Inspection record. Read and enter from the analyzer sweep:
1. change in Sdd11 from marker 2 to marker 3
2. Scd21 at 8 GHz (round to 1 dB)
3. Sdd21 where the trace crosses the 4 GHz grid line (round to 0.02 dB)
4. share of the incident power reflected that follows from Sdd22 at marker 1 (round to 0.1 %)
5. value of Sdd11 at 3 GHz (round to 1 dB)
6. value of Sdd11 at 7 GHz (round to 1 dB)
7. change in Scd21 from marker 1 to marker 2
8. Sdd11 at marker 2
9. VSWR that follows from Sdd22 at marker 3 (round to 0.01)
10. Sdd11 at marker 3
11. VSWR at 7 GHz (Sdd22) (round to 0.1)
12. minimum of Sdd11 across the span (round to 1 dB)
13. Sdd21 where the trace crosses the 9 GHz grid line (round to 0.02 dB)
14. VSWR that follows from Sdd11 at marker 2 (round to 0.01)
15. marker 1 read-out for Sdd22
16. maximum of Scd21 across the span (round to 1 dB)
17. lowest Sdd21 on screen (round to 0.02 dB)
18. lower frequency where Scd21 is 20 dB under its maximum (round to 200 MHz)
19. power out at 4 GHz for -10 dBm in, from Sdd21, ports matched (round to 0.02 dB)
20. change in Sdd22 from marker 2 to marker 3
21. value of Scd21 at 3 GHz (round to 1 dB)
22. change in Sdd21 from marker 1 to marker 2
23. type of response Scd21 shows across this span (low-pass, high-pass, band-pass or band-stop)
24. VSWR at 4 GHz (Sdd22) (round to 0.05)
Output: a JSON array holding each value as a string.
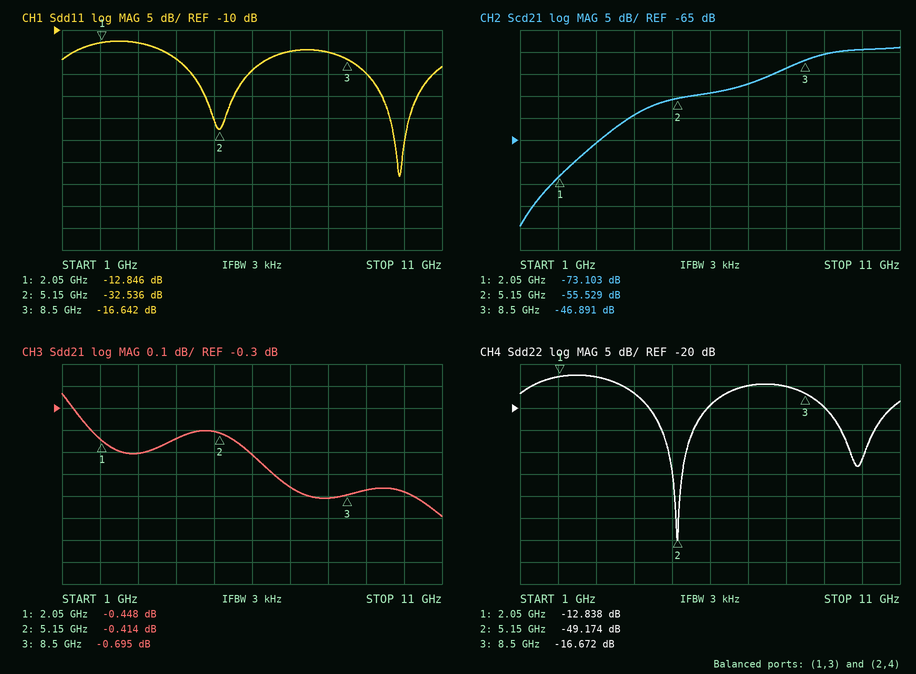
["15.894 dB", "-49 dB", "-0.44 dB", "5.2 %", "-13 dB", "-15 dB", "17.574 dB", "-32.536 dB", "1.34", "-16.642 dB", "1.4", "-43 dB", "-0.68 dB", "1.05", "-12.838 dB", "-44 dB", "-0.80 dB", "3.2 GHz", "-10.44 dBm", "32.502 dB", "-66 dB", "0.034 dB", "high-pass", "1.35"]
